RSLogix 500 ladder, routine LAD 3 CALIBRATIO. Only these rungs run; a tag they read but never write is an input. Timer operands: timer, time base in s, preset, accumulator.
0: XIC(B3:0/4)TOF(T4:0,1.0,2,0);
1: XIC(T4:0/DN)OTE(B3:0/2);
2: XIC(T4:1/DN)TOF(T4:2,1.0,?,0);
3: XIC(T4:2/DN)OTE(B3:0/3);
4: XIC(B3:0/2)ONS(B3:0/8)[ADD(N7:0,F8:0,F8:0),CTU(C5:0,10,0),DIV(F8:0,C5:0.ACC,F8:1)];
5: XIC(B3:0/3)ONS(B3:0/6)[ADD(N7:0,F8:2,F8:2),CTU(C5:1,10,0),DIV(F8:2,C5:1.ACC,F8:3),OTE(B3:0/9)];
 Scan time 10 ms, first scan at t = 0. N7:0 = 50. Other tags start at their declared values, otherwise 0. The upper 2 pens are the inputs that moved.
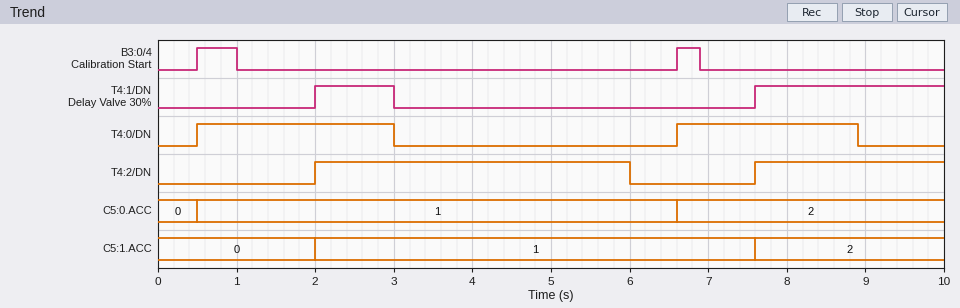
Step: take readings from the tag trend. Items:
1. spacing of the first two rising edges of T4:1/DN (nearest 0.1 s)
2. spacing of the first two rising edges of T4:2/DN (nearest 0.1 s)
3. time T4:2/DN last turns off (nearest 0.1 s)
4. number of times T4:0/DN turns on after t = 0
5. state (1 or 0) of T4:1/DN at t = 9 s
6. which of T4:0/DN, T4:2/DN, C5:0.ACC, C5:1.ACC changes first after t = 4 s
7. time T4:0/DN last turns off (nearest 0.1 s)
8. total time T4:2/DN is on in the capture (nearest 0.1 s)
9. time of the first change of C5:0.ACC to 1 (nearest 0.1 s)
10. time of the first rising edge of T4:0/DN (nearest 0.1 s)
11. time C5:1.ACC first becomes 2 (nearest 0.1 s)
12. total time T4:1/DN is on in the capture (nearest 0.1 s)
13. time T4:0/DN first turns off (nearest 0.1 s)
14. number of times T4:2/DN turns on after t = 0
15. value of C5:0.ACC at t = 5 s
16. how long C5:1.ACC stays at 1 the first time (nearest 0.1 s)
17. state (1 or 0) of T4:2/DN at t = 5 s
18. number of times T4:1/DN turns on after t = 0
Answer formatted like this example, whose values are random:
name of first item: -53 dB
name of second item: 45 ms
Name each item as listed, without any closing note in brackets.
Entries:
spacing of the first two rising edges of T4:1/DN: 5.6 s
spacing of the first two rising edges of T4:2/DN: 5.6 s
time T4:2/DN last turns off: 6.0 s
number of times T4:0/DN turns on after t = 0: 2
state (1 or 0) of T4:1/DN at t = 9 s: 1
which of T4:0/DN, T4:2/DN, C5:0.ACC, C5:1.ACC changes first after t = 4 s: T4:2/DN
time T4:0/DN last turns off: 8.9 s
total time T4:2/DN is on in the capture: 6.4 s
time of the first change of C5:0.ACC to 1: 0.5 s
time of the first rising edge of T4:0/DN: 0.5 s
time C5:1.ACC first becomes 2: 7.6 s
total time T4:1/DN is on in the capture: 3.4 s
time T4:0/DN first turns off: 3.0 s
number of times T4:2/DN turns on after t = 0: 2
value of C5:0.ACC at t = 5 s: 1
how long C5:1.ACC stays at 1 the first time: 5.6 s
state (1 or 0) of T4:2/DN at t = 5 s: 1
number of times T4:1/DN turns on after t = 0: 2
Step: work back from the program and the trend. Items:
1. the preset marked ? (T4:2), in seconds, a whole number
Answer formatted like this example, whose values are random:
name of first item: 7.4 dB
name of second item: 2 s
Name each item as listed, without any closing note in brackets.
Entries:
the preset marked ? (T4:2), in seconds, a whole number: 3 s
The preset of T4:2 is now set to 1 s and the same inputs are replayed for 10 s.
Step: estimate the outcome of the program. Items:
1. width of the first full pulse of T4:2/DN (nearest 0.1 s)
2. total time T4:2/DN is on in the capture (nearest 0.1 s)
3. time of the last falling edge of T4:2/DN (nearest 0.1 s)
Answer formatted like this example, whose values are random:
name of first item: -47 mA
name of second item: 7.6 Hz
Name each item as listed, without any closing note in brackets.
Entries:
width of the first full pulse of T4:2/DN: 2.0 s
total time T4:2/DN is on in the capture: 4.4 s
time of the last falling edge of T4:2/DN: 4.0 s
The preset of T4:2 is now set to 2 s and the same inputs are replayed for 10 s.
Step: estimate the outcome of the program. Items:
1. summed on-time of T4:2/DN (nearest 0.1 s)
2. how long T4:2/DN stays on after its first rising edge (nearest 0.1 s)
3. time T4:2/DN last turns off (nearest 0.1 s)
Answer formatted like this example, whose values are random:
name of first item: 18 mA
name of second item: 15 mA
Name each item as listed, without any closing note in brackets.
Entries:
summed on-time of T4:2/DN: 5.4 s
how long T4:2/DN stays on after its first rising edge: 3.0 s
time T4:2/DN last turns off: 5.0 s
